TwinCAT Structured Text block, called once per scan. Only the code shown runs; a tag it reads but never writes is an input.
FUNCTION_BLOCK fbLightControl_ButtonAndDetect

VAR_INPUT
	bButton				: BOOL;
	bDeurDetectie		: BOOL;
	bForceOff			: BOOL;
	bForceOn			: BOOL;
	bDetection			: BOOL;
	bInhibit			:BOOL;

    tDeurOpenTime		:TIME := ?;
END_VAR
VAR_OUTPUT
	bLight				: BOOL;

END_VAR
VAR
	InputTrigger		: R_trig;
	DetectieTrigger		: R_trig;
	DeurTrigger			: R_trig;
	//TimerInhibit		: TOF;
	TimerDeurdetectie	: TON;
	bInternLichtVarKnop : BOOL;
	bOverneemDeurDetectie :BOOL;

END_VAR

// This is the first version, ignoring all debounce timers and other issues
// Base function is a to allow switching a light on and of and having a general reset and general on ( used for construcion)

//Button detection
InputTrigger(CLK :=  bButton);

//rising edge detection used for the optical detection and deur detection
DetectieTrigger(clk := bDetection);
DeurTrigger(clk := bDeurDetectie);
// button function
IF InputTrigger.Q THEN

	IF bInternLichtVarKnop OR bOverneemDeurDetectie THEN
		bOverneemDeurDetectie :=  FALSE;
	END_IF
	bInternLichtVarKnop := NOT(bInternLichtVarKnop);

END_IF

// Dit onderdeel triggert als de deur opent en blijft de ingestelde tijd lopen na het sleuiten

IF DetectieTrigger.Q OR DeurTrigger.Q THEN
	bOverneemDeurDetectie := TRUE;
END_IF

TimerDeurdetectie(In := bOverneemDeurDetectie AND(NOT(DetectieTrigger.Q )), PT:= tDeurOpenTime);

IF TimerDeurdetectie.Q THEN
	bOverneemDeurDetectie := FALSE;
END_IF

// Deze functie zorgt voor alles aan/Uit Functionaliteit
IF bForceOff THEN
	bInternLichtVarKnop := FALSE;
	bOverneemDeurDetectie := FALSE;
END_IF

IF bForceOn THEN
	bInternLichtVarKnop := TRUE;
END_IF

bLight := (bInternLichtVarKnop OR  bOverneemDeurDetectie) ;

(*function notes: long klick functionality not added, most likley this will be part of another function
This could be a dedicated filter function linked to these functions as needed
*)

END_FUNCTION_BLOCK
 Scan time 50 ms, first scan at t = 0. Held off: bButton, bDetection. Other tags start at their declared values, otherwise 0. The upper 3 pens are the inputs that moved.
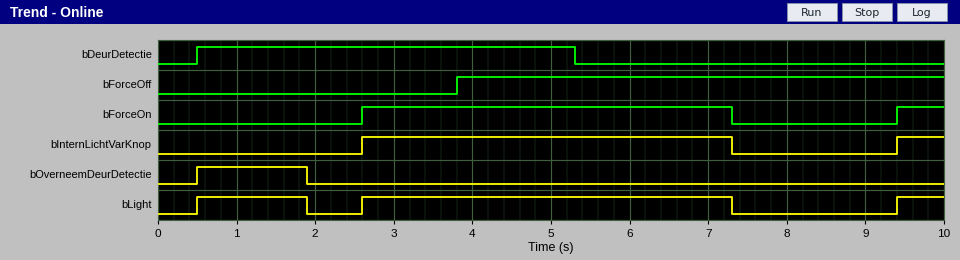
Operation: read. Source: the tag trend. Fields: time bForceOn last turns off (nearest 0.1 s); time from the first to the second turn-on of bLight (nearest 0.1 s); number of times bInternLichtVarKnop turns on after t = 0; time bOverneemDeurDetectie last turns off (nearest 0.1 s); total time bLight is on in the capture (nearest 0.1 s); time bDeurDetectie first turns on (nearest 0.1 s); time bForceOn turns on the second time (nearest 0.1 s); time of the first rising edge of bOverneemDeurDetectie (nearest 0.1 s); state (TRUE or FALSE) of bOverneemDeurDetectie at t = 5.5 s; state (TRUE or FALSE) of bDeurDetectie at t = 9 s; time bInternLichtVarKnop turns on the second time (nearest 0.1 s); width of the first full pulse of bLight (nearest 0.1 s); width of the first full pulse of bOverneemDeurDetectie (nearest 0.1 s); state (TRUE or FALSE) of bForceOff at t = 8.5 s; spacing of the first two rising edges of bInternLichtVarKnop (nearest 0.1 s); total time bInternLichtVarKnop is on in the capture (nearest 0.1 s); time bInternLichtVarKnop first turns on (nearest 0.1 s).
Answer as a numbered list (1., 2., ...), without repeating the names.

1. 7.3 s
2. 2.1 s
3. 2
4. 1.9 s
5. 6.7 s
6. 0.5 s
7. 9.4 s
8. 0.5 s
9. FALSE
10. FALSE
11. 9.4 s
12. 1.4 s
13. 1.4 s
14. TRUE
15. 6.8 s
16. 5.3 s
17. 2.6 s
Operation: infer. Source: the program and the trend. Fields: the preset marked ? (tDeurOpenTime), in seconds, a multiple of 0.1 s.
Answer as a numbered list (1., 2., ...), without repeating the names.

1. 1.4 s
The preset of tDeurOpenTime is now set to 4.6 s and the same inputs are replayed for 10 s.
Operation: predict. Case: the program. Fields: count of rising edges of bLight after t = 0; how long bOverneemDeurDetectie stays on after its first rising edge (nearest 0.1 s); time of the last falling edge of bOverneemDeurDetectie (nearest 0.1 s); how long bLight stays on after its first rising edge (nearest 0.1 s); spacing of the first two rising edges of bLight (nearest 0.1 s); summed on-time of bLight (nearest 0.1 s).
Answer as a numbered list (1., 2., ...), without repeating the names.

1. 2
2. 3.3 s
3. 3.8 s
4. 6.8 s
5. 8.9 s
6. 7.4 s
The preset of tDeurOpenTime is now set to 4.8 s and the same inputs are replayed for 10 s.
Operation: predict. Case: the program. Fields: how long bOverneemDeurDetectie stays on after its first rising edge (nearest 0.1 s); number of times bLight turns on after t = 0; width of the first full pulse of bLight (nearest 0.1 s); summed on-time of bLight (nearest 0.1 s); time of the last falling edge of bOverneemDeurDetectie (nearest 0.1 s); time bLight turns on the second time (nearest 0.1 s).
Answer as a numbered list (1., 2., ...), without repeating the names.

1. 3.3 s
2. 2
3. 6.8 s
4. 7.4 s
5. 3.8 s
6. 9.4 s
